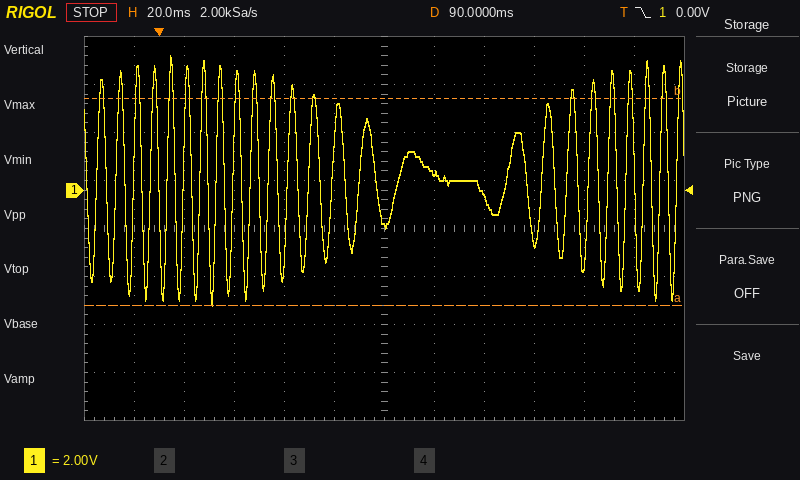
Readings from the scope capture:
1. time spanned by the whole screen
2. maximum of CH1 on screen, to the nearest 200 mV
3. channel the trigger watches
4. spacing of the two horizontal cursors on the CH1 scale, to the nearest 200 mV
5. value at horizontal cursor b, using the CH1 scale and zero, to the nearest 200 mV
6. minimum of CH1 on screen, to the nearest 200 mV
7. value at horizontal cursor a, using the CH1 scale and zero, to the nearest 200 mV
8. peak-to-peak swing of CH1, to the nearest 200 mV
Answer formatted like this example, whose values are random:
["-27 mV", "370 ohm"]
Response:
["240 ms", "5.6 V", "CH1", "8.6 V", "3.8 V", "-4.8 V", "-4.8 V", "10.4 V"]
